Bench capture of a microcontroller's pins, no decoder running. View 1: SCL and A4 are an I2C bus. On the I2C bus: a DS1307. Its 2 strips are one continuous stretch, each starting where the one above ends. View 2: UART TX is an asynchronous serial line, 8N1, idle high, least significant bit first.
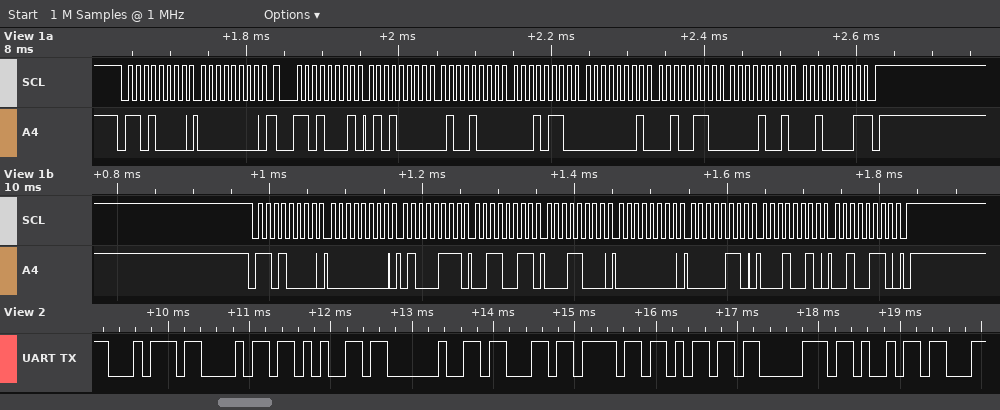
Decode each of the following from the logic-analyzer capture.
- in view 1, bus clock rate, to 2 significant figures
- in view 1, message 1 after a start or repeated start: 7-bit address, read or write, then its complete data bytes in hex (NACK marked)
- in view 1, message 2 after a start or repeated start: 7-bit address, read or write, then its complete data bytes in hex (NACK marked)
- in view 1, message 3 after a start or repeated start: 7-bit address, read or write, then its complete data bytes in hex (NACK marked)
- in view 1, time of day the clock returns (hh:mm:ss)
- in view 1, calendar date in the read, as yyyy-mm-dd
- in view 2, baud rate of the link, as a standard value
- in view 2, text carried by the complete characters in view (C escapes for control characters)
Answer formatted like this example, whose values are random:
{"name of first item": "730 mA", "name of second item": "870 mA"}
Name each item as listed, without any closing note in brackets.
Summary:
{"in view 1, bus clock rate, to 2 significant figures": "100 kHz", "in view 1, message 1 after a start or repeated start: 7-bit address, read or write, then its complete data bytes in hex": "0x68 write: 00", "in view 1, message 2 after a start or repeated start: 7-bit address, read or write, then its complete data bytes in hex": "0x68 read: 50 48 16 01 26 09 21 NACK", "in view 1, message 3 after a start or repeated start: 7-bit address, read or write, then its complete data bytes in hex": "0x68 write: 00 47 33 18 00 06 12 26", "in view 1, time of day the clock returns": "16:48:50", "in view 1, calendar date in the read, as yyyy-mm-dd": "2021-09-26", "in view 2, baud rate of the link, as a standard value": "9600 baud", "in view 2, text carried by the complete characters in view": "\"the compi\""}
